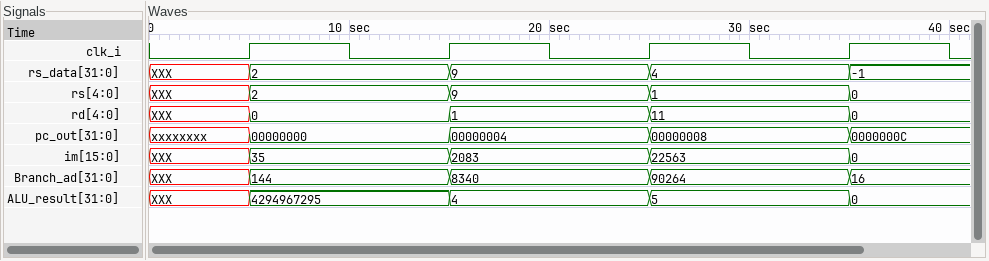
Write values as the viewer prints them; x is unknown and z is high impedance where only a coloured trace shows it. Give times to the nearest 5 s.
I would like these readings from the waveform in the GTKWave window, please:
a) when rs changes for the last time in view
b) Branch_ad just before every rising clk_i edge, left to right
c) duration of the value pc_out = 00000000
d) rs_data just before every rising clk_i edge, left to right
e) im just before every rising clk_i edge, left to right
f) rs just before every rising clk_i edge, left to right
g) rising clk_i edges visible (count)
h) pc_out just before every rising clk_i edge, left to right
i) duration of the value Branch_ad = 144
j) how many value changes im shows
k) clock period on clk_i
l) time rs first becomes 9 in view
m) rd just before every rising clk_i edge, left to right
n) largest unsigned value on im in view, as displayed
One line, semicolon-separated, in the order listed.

35 s; XXX, 144, 8340, 90264; 10 s; XXX, 2, 9, 4; XXX, 35, 2083, 22563; XXX, 2, 9, 1; 4; xxxxxxxx, 00000000, 00000004, 00000008; 10 s; 4; 10 s; 15 s; XXX, 0, 1, 11; 22563
